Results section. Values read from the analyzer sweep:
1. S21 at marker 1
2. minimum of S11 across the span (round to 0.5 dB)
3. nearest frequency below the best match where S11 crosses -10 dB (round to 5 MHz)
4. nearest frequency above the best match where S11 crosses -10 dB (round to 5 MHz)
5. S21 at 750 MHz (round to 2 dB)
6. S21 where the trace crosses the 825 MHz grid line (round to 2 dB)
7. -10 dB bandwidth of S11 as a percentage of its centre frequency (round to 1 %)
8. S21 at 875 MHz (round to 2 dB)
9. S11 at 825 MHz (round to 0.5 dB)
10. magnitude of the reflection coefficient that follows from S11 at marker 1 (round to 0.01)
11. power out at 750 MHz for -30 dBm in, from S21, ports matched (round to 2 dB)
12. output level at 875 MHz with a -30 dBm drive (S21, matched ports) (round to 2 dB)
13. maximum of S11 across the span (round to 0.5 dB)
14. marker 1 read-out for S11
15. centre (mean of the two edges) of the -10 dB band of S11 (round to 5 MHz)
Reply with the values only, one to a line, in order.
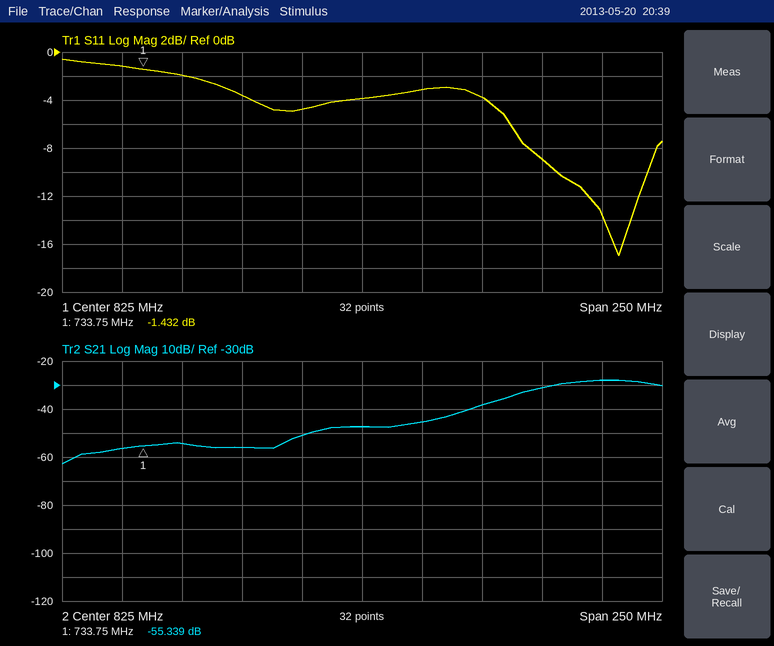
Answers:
-55.339 dB
-17.0 dB
905 MHz
945 MHz
-54 dB
-48 dB
4 %
-38 dB
-4.0 dB
0.85
-84 dBm
-68 dBm
-0.5 dB
-1.432 dB
925 MHz
